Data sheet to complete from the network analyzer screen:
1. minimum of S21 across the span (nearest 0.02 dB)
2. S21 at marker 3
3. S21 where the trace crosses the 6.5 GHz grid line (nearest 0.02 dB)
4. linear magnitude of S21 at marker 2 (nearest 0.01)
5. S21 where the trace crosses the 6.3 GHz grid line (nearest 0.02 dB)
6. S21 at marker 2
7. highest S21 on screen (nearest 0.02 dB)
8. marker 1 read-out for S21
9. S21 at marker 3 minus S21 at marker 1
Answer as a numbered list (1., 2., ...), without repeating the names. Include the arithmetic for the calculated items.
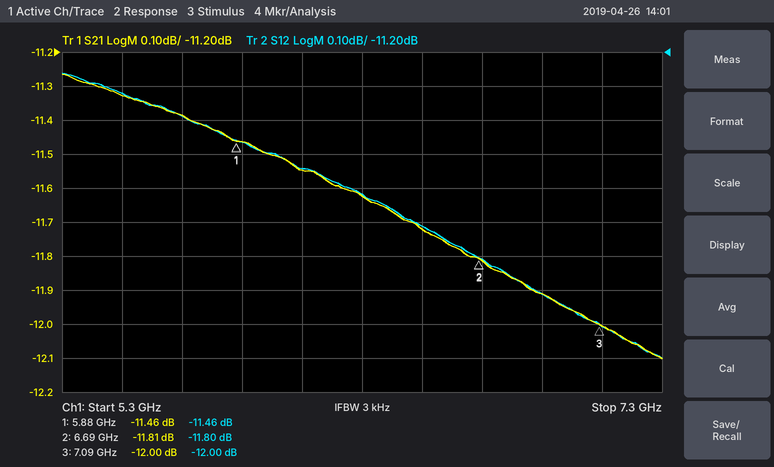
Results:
1. -12.10 dB
2. -12.00 dB
3. -11.72 dB
4. 10^(-11.81/20) ≈ 0.26
5. -11.62 dB
6. -11.81 dB
7. -11.26 dB
8. -11.46 dB
9. -12 − (-11.46) = -0.54 dB
